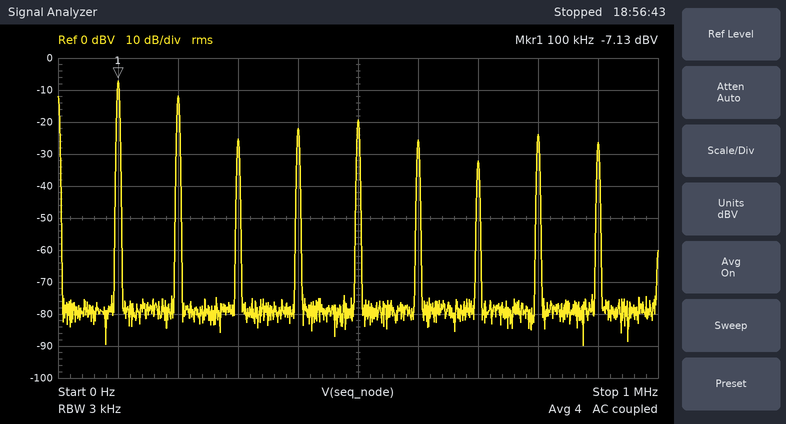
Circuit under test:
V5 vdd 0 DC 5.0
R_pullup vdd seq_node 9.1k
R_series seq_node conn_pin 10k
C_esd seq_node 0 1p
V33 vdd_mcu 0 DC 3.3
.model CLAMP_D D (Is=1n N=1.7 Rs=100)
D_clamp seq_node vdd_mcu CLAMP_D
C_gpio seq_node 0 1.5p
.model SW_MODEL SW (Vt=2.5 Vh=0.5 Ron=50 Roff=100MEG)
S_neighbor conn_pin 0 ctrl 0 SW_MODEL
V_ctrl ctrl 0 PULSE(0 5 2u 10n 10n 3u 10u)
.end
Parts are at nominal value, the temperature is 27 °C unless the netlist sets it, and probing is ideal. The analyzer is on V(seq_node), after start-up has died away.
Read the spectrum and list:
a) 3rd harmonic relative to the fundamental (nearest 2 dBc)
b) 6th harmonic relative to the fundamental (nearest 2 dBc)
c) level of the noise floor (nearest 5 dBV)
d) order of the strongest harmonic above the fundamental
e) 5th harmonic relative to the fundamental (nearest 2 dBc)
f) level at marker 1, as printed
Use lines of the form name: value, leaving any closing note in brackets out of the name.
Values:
3rd harmonic relative to the fundamental: -18 dBc
6th harmonic relative to the fundamental: -18 dBc
level of the noise floor: -80 dBV
order of the strongest harmonic above the fundamental: 2
5th harmonic relative to the fundamental: -12 dBc
level at marker 1, as printed: -7.13 dBV
